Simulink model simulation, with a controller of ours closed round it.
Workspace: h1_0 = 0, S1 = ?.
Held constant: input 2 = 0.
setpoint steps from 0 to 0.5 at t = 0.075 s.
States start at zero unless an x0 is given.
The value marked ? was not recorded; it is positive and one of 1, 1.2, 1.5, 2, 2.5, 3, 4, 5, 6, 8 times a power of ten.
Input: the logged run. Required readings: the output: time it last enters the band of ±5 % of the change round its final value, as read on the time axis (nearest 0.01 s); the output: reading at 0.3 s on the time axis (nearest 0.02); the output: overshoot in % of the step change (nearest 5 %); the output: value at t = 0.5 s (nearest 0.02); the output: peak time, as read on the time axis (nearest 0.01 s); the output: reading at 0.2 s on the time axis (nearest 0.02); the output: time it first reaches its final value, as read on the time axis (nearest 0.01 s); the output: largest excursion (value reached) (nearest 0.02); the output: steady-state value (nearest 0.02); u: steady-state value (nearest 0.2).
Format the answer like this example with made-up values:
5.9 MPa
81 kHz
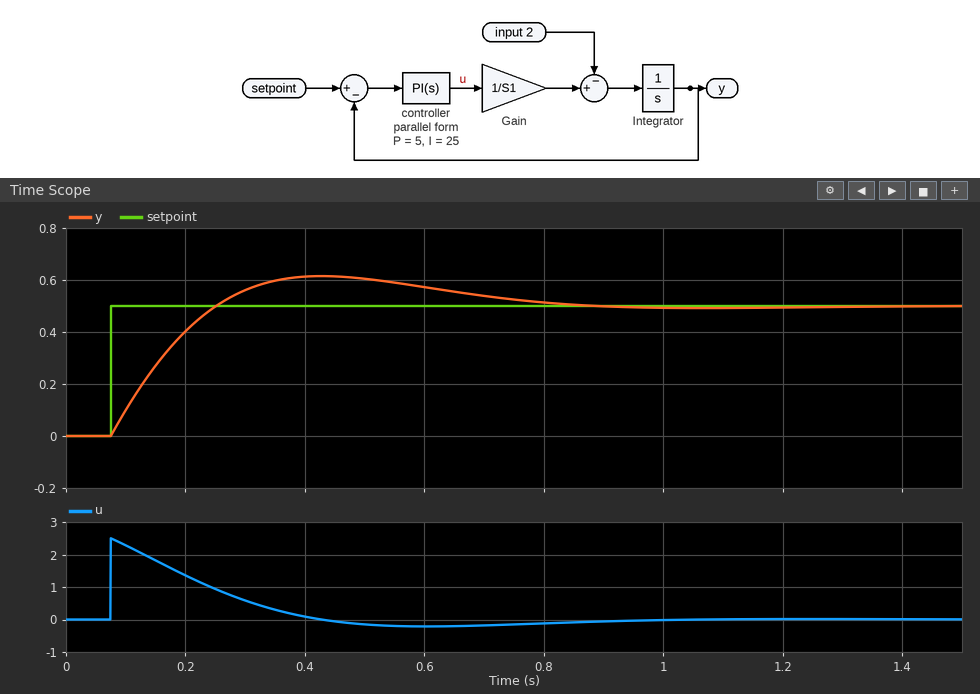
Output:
0.75 s
0.56
25 %
0.60
0.43 s
0.40
0.25 s
0.62
0.50
0.0
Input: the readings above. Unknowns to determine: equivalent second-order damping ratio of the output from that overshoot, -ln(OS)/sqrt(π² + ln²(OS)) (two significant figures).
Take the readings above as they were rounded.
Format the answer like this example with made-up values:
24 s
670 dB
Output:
0.40
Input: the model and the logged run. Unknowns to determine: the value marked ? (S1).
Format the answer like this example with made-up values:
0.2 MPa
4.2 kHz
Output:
0.6
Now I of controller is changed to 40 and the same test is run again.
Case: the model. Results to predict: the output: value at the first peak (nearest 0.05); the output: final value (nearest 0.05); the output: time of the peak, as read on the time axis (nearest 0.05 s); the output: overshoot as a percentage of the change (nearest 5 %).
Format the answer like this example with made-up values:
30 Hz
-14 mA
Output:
0.65
0.50
0.35 s
30 %
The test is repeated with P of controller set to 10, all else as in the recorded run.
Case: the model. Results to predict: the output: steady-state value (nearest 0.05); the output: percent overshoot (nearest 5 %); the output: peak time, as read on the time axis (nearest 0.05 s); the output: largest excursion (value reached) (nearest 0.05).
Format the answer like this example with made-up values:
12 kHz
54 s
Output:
0.50
10 %
0.35 s
0.55
